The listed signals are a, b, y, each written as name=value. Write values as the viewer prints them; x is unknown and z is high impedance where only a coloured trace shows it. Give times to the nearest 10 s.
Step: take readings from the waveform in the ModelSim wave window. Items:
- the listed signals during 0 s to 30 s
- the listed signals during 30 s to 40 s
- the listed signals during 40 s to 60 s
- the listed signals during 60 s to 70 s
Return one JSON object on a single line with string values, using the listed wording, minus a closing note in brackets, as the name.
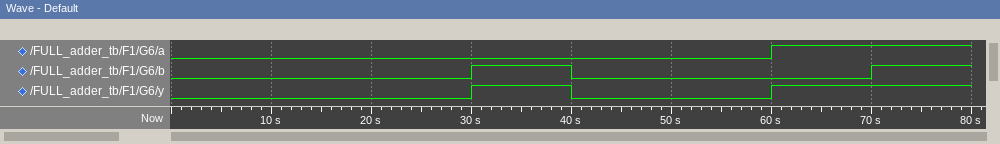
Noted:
{"the listed signals during 0 s to 30 s": "a=0, b=0, y=0", "the listed signals during 30 s to 40 s": "a=0, b=1, y=1", "the listed signals during 40 s to 60 s": "a=0, b=0, y=0", "the listed signals during 60 s to 70 s": "a=1, b=0, y=1"}
